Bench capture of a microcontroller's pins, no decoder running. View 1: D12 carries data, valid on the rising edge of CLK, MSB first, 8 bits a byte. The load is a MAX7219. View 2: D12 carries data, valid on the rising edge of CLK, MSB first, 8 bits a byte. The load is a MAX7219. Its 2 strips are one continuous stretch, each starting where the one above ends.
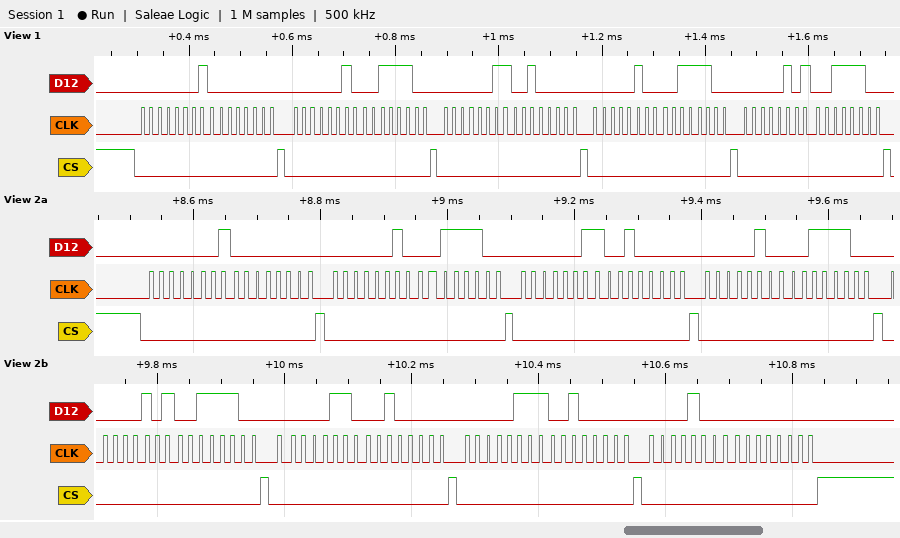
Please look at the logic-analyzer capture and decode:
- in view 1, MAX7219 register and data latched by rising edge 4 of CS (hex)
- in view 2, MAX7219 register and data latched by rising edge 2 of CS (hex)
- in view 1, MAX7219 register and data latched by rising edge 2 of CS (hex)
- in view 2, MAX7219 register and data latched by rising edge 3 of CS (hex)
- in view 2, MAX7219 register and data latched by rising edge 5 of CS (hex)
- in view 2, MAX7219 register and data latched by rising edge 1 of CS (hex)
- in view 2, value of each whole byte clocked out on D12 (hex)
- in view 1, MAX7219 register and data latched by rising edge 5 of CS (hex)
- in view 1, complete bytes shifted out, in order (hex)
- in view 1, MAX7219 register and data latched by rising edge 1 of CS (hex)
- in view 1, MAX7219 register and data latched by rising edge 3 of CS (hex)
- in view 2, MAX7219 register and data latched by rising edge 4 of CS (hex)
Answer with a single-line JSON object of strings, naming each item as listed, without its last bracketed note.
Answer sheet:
{"in view 1, MAX7219 register and data latched by rising edge 4 of CS": "register 0x4, data 0x3C", "in view 2, MAX7219 register and data latched by rising edge 2 of CS": "register 0x2, data 0x3C", "in view 1, MAX7219 register and data latched by rising edge 2 of CS": "register 0x2, data 0x3C", "in view 2, MAX7219 register and data latched by rising edge 3 of CS": "register 0x3, data 0x20", "in view 2, MAX7219 register and data latched by rising edge 5 of CS": "register 0x5, data 0x3C", "in view 2, MAX7219 register and data latched by rising edge 1 of CS": "register 0x1, data 0x00", "in view 2, value of each whole byte clocked out on D12": "01 00 02 3C 03 20 04 3C 05 3C 06 20 07 20 08 00", "in view 1, MAX7219 register and data latched by rising edge 5 of CS": "register 0x5, data 0x3C", "in view 1, complete bytes shifted out, in order": "0x01 0x00 0x02 0x3C 0x03 0x20 0x04 0x3C 0x05 0x3C", "in view 1, MAX7219 register and data latched by rising edge 1 of CS": "register 0x1, data 0x00", "in view 1, MAX7219 register and data latched by rising edge 3 of CS": "register 0x3, data 0x20", "in view 2, MAX7219 register and data latched by rising edge 4 of CS": "register 0x4, data 0x3C"}
